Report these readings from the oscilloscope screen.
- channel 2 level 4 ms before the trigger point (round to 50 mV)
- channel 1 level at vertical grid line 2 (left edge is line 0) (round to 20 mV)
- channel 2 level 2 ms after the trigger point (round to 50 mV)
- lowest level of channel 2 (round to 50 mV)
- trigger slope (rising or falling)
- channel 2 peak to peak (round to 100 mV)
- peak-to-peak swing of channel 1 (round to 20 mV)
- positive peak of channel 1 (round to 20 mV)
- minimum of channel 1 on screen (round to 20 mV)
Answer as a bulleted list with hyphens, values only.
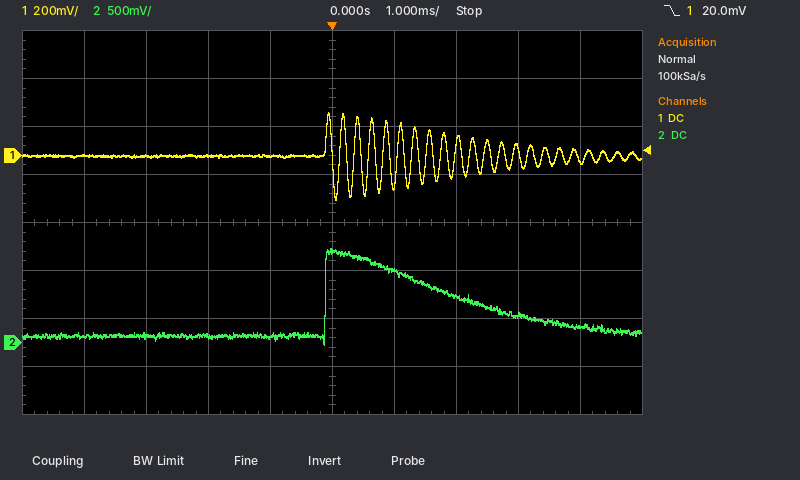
- 50 mV
- 0 mV
- 500 mV
- 0 mV
- falling
- 1.00 V
- 360 mV
- 180 mV
- -180 mV
